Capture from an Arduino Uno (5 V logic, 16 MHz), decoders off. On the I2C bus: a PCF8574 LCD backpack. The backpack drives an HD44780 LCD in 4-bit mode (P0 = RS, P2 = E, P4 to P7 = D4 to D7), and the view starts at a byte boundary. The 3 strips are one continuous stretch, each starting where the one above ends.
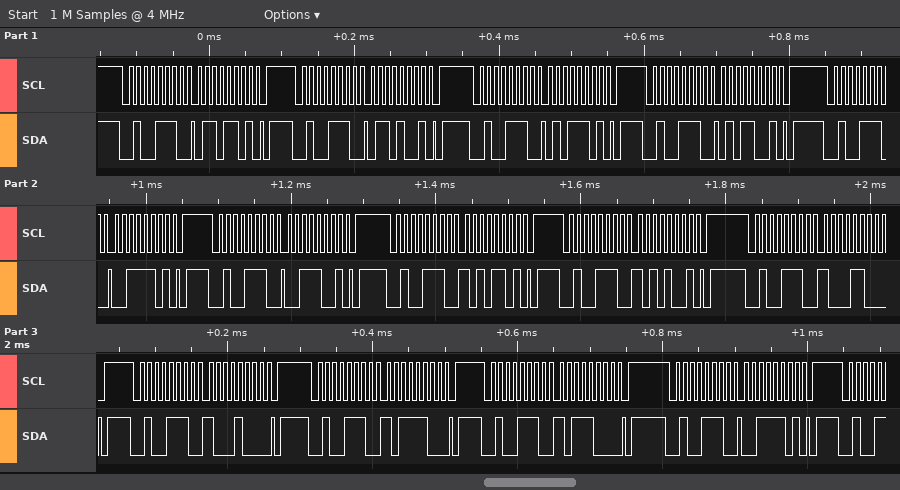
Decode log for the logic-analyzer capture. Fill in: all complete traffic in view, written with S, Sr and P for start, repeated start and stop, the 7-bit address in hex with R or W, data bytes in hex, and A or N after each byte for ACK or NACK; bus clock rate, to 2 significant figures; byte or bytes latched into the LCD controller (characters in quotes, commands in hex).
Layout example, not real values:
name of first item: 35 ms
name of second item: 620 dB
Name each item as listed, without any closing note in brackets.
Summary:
all complete traffic in view, written with S, Sr and P for start, repeated start and stop, the 7-bit address in hex with R or W, data bytes in hex, and A or N after each byte for ACK or NACK: S 27W A 6D A P S 27W A 69 A P S 27W A 5D A P S 27W A 59 A P S 27W A 3D A P S 27W A 39 A P S 27W A AD A P S 27W A A9 A P S 27W A 8C A P S 27W A 88 A P S 27W A BC A P S 27W A B8 A P S 27W A 3D A P
bus clock rate, to 2 significant figures: 100 kHz
byte or bytes latched into the LCD controller: 'e' ':' 0x8B
